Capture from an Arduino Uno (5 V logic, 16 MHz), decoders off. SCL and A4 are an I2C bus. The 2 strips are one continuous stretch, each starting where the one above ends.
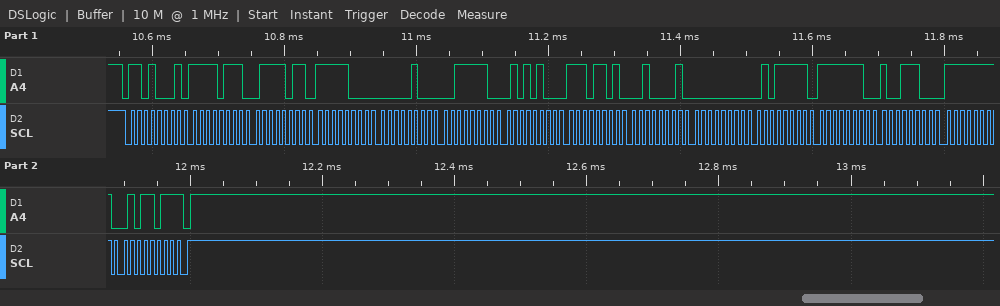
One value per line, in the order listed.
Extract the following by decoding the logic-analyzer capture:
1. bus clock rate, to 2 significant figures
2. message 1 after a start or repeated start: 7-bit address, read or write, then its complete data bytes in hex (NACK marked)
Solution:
100 kHz
0x68 read: F7 7B F8 04 3E 54 ED 21 00 5F FE 9C FF 5B NACK
